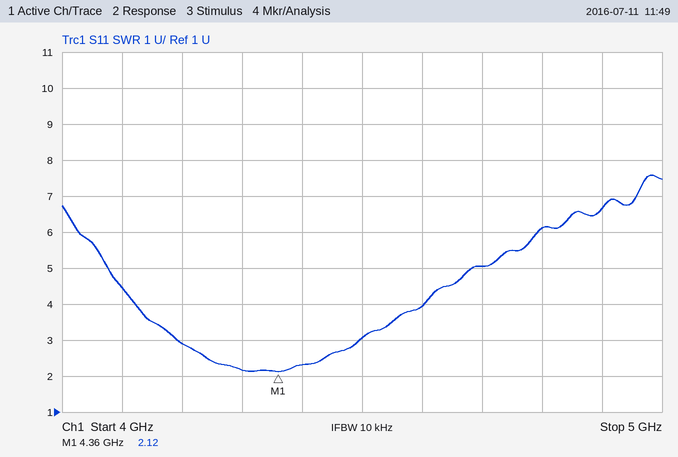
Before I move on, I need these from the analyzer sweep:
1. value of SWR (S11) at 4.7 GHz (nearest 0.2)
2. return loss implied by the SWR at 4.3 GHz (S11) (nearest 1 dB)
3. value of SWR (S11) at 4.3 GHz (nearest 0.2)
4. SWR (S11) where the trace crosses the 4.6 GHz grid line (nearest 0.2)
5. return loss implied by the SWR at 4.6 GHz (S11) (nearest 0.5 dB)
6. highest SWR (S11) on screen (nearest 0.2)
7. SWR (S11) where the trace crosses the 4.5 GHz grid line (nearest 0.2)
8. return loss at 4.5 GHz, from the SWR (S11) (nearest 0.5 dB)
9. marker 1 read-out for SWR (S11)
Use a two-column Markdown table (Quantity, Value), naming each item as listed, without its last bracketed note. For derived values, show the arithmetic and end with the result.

| Quantity | Value |
|---|---|
| value of SWR (S11) at 4.7 GHz | 5.0 |
| return loss implied by the SWR at 4.3 GHz (S11) | −20 log10((2.2 − 1)/(2.2 + 1)) ≈ 9 dB |
| value of SWR (S11) at 4.3 GHz | 2.2 |
| SWR (S11) where the trace crosses the 4.6 GHz grid line | 4.0 |
| return loss implied by the SWR at 4.6 GHz (S11) | −20 log10((4 − 1)/(4 + 1)) ≈ 4.44 dB, so 4.5 dB to the nearest 0.5 dB |
| highest SWR (S11) on screen | 7.6 |
| SWR (S11) where the trace crosses the 4.5 GHz grid line | 3.0 |
| return loss at 4.5 GHz, from the SWR (S11) | −20 log10((3 − 1)/(3 + 1)) ≈ 6.0 dB |
| marker 1 read-out for SWR | 2.12 |
